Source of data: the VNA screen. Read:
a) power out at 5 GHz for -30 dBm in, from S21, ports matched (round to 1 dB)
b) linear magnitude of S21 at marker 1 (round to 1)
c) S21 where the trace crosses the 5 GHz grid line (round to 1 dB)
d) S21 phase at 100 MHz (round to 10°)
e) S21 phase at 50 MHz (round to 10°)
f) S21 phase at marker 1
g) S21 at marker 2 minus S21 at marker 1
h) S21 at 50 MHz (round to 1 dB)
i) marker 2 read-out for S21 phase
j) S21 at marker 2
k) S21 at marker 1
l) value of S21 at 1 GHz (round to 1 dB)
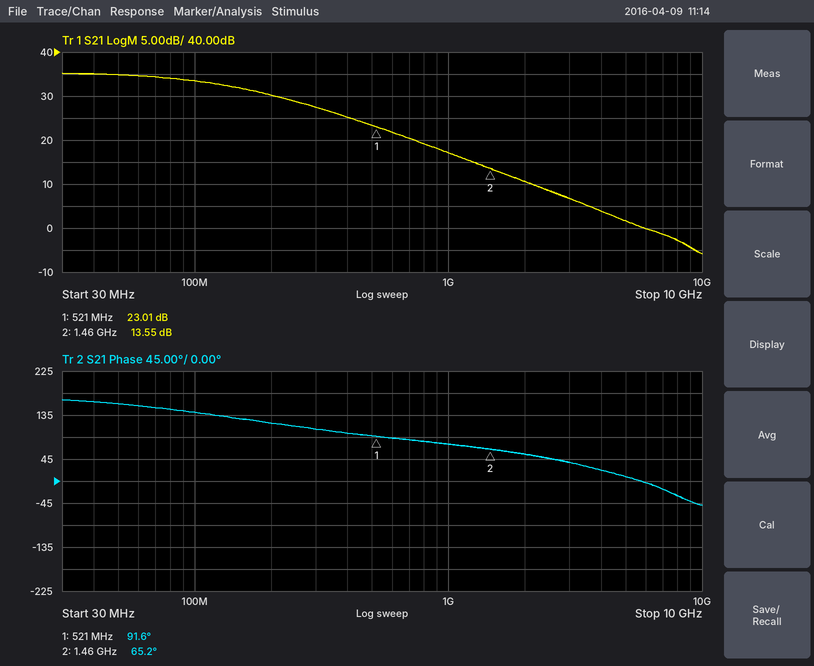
-28 dBm
14
2 dB
140°
160°
91.6°
-9.46 dB
35 dB
65.2°
13.55 dB
23.01 dB
17 dB
